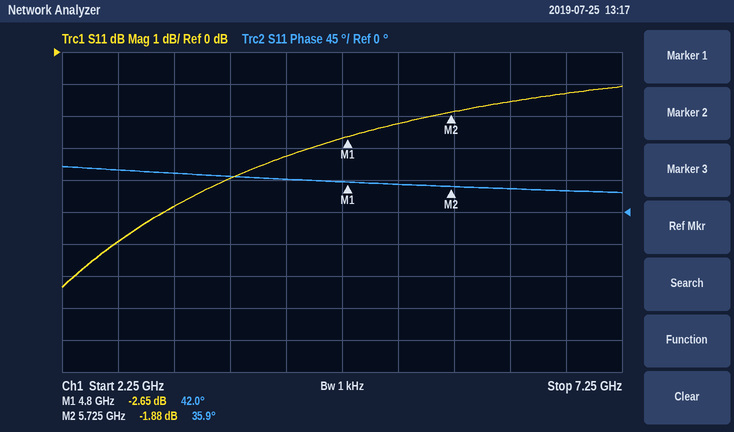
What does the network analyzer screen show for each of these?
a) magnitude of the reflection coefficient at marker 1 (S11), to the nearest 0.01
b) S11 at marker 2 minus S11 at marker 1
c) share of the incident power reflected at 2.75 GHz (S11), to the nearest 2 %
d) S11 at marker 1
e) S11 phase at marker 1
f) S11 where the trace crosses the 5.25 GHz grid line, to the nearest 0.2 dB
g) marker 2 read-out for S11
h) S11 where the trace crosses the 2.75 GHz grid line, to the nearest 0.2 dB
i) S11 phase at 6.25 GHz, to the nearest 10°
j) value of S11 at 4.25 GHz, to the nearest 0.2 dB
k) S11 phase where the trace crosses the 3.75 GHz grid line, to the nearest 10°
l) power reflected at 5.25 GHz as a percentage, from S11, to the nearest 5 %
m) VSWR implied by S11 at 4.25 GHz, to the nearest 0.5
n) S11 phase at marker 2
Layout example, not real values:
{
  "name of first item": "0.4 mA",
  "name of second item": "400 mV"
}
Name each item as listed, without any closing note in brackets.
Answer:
{
  "magnitude of the reflection coefficient at marker 1 (S11), to the nearest 0.01": "0.74",
  "S11 at marker 2 minus S11 at marker 1": "0.77 dB",
  "share of the incident power reflected at 2.75 GHz (S11), to the nearest 2 %": "26 %",
  "S11 at marker 1": "-2.65 dB",
  "S11 phase at marker 1": "42.0°",
  "S11 where the trace crosses the 5.25 GHz grid line, to the nearest 0.2 dB": "-2.2 dB",
  "marker 2 read-out for S11": "-1.88 dB",
  "S11 where the trace crosses the 2.75 GHz grid line, to the nearest 0.2 dB": "-6.0 dB",
  "S11 phase at 6.25 GHz, to the nearest 10°": "30°",
  "value of S11 at 4.25 GHz, to the nearest 0.2 dB": "-3.2 dB",
  "S11 phase where the trace crosses the 3.75 GHz grid line, to the nearest 10°": "50°",
  "power reflected at 5.25 GHz as a percentage, from S11, to the nearest 5 %": "60 %",
  "VSWR implied by S11 at 4.25 GHz, to the nearest 0.5": "5.5",
  "S11 phase at marker 2": "35.9°"
}
